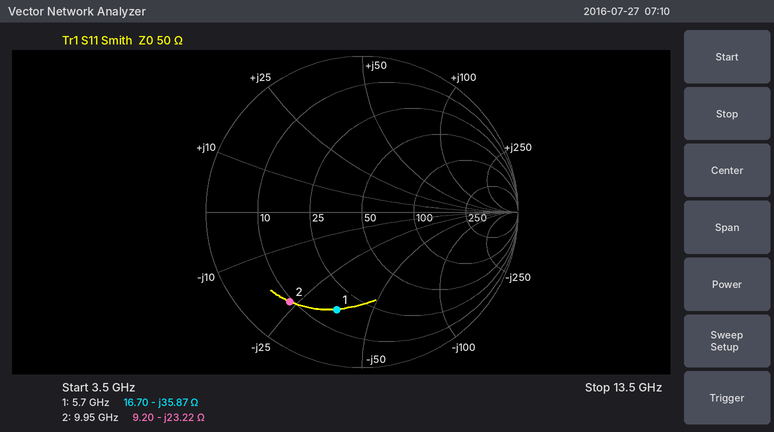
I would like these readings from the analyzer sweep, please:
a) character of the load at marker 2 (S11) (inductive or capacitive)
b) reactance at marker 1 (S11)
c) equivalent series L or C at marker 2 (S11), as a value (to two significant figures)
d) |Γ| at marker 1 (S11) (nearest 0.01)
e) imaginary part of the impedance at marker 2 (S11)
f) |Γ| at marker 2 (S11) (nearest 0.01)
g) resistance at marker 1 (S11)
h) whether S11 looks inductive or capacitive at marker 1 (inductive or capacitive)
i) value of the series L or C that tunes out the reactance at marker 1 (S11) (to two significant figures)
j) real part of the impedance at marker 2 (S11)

capacitive
-35.87 Ω
690 fF
0.65
-23.22 Ω
0.74
16.70 Ω
capacitive
1.0 nH
9.20 Ω
